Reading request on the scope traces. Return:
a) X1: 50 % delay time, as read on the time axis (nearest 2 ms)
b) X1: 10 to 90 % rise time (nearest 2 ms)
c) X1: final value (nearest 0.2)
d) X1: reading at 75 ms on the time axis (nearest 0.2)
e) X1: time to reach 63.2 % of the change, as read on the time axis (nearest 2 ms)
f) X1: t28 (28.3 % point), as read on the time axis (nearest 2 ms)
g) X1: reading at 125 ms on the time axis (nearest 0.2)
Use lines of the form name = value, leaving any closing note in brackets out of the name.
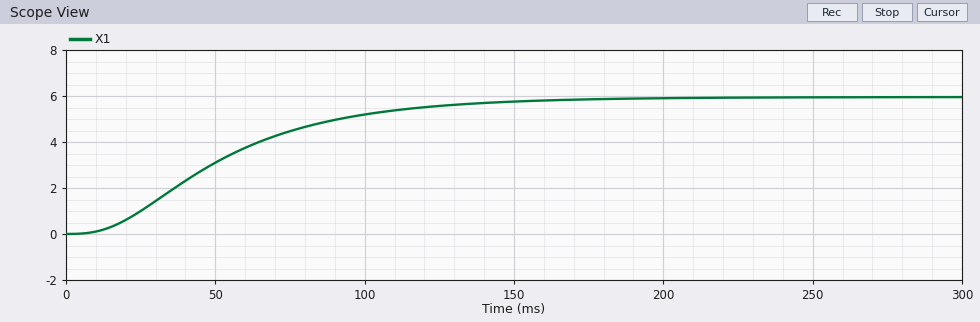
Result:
X1: 50 % delay time, as read on the time axis = 48 ms
X1: 10 to 90 % rise time = 90 ms
X1: final value = 6.0
X1: reading at 75 ms on the time axis = 4.4
X1: time to reach 63.2 % of the change, as read on the time axis = 60 ms
X1: t28 (28.3 % point), as read on the time axis = 32 ms
X1: reading at 125 ms on the time axis = 5.6
